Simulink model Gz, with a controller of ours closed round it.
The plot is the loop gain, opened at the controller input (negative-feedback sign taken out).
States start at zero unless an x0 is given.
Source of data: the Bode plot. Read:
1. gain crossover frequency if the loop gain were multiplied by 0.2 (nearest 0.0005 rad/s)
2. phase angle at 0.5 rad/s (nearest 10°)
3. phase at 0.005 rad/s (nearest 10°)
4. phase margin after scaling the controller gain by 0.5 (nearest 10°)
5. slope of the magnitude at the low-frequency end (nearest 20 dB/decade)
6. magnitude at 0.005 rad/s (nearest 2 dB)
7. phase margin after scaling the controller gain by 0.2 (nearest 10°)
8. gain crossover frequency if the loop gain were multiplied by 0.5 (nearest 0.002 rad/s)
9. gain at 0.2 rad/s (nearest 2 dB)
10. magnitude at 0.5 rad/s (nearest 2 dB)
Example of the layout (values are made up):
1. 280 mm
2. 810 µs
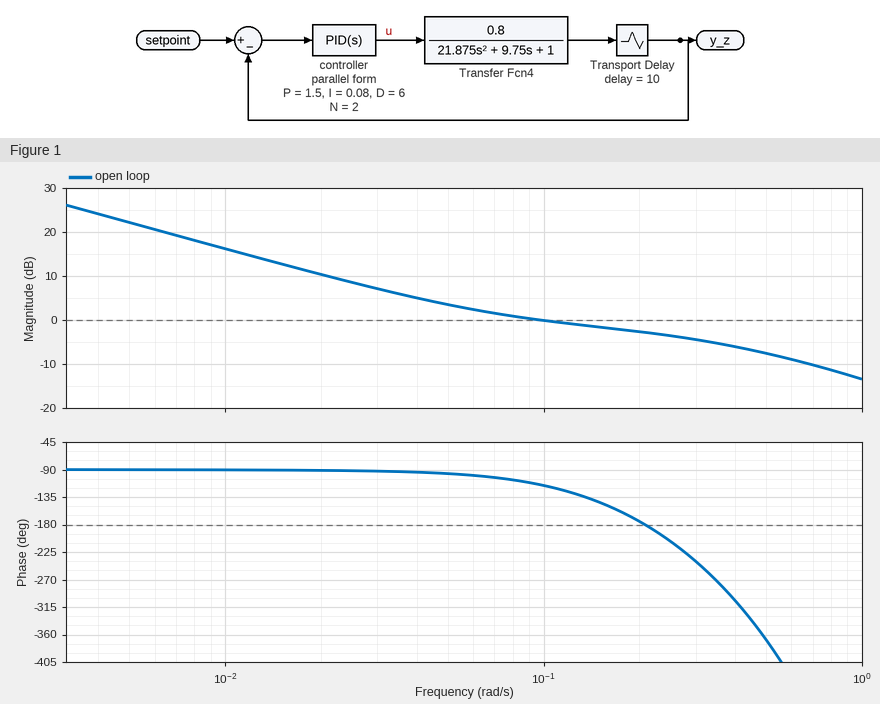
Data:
1. 0.0130 rad/s
2. -370°
3. -90°
4. 90°
5. -20 dB/decade
6. 22 dB
7. 90°
8. 0.034 rad/s
9. -2 dB
10. -8 dB
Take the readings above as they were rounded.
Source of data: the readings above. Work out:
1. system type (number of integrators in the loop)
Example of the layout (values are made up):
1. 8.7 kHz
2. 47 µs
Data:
1. 1
